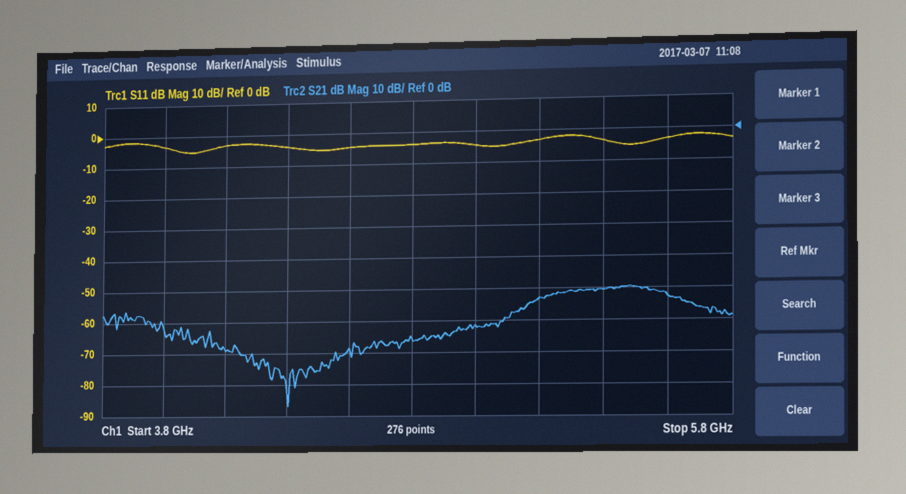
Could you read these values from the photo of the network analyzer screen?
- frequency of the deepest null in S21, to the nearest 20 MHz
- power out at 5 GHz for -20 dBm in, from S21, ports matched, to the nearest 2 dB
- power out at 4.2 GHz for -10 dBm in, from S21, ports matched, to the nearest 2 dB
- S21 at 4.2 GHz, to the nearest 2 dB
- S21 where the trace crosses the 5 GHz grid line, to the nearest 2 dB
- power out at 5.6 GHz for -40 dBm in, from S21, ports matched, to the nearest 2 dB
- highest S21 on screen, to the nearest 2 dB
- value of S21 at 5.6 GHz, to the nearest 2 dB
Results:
4.40 GHz
-82 dBm
-78 dBm
-68 dB
-62 dB
-92 dBm
-50 dB
-52 dB
